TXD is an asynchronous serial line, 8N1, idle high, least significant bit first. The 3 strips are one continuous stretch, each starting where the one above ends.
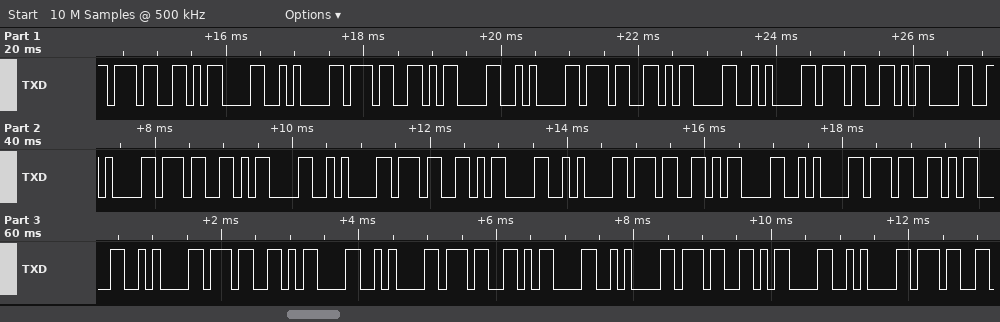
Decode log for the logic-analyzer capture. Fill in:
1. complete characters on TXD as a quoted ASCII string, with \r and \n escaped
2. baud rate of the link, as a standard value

"7\r\n7\r\n7\r\n7\r\n7\r\n7\r\n7\r\n7\r\n7\r\n7\r\n7\r\n7"
9600 baud
